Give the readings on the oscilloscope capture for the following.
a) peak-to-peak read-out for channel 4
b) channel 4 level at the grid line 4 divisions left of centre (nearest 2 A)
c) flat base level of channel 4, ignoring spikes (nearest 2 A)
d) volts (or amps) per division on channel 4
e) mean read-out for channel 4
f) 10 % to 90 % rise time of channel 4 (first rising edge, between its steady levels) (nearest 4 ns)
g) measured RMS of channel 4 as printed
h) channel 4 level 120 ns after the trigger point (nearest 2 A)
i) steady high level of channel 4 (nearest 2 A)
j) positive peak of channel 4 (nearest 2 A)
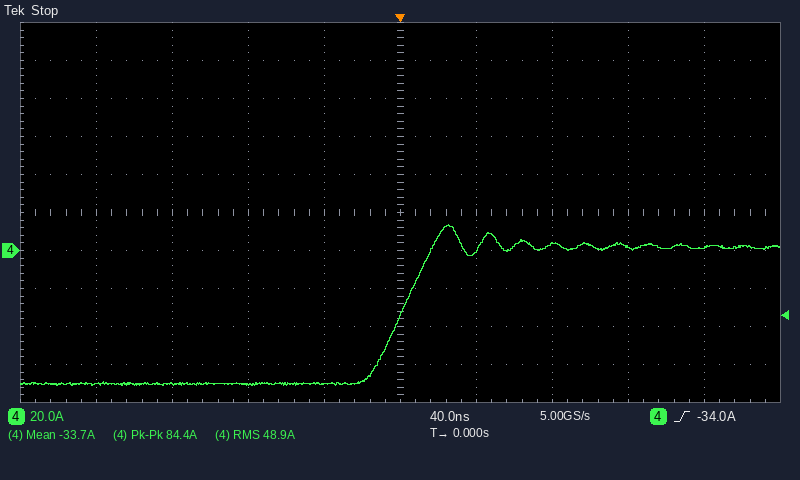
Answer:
84.4 A
-70 A
-70 A
20 A
-33.7 A
28 ns
48.9 A
2 A
2 A
14 A
